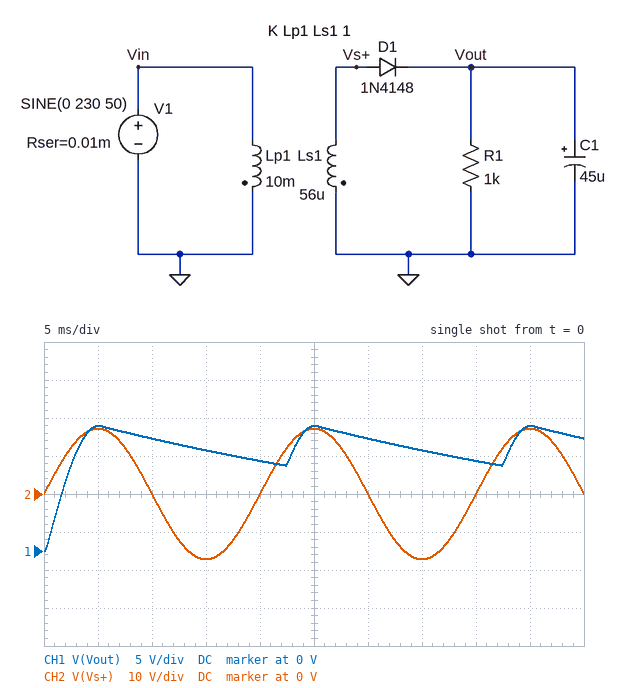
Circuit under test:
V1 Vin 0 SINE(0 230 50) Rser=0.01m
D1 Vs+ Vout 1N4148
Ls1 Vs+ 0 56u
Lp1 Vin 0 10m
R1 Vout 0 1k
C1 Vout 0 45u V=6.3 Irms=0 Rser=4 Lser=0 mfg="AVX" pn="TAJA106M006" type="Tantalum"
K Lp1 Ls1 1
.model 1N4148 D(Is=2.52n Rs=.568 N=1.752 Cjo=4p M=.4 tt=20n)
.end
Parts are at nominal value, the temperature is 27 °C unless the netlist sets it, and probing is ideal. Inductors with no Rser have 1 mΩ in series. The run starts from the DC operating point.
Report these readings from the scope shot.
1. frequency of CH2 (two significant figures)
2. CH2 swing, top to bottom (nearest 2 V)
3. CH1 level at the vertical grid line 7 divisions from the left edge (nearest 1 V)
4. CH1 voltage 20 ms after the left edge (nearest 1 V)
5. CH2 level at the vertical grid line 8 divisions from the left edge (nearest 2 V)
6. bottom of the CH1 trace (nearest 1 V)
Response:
50 Hz
34 V
13 V
12 V
0 V
0 V
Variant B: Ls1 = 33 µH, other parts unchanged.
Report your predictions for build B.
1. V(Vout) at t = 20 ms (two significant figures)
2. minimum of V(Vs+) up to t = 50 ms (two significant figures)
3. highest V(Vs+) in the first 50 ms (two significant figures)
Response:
9.0 V
-13 V
13 V
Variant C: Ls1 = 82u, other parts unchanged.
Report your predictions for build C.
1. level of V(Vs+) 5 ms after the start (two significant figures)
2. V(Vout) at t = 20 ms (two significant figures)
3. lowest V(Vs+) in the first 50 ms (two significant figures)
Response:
21 V
14 V
-21 V
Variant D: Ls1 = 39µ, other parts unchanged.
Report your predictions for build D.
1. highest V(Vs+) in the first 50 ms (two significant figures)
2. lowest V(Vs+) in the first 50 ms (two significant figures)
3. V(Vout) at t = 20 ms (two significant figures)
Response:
14 V
-14 V
9.8 V
